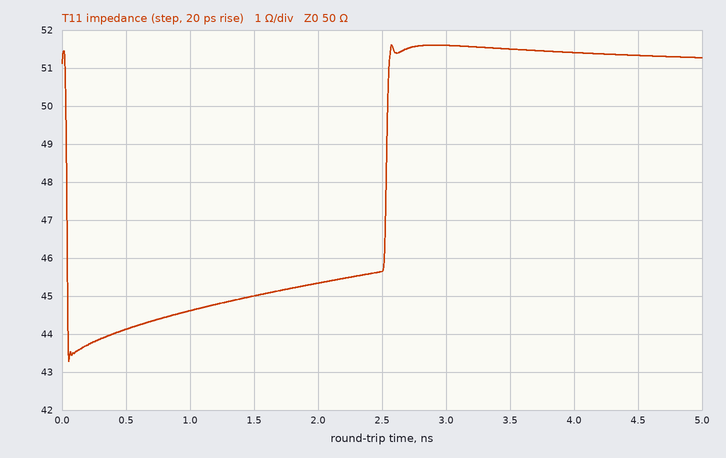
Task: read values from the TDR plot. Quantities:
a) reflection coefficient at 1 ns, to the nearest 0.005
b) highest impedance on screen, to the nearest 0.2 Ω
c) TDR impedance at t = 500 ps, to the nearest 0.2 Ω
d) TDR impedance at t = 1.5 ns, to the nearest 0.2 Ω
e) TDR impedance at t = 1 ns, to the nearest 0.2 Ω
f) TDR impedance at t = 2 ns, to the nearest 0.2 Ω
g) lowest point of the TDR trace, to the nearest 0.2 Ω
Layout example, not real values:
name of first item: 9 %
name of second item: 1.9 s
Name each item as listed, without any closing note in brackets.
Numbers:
reflection coefficient at 1 ns, to the nearest 0.005: -0.055
highest impedance on screen, to the nearest 0.2 Ω: 51.6 Ω
TDR impedance at t = 500 ps, to the nearest 0.2 Ω: 44.2 Ω
TDR impedance at t = 1.5 ns, to the nearest 0.2 Ω: 45.0 Ω
TDR impedance at t = 1 ns, to the nearest 0.2 Ω: 44.6 Ω
TDR impedance at t = 2 ns, to the nearest 0.2 Ω: 45.4 Ω
lowest point of the TDR trace, to the nearest 0.2 Ω: 43.2 Ω
